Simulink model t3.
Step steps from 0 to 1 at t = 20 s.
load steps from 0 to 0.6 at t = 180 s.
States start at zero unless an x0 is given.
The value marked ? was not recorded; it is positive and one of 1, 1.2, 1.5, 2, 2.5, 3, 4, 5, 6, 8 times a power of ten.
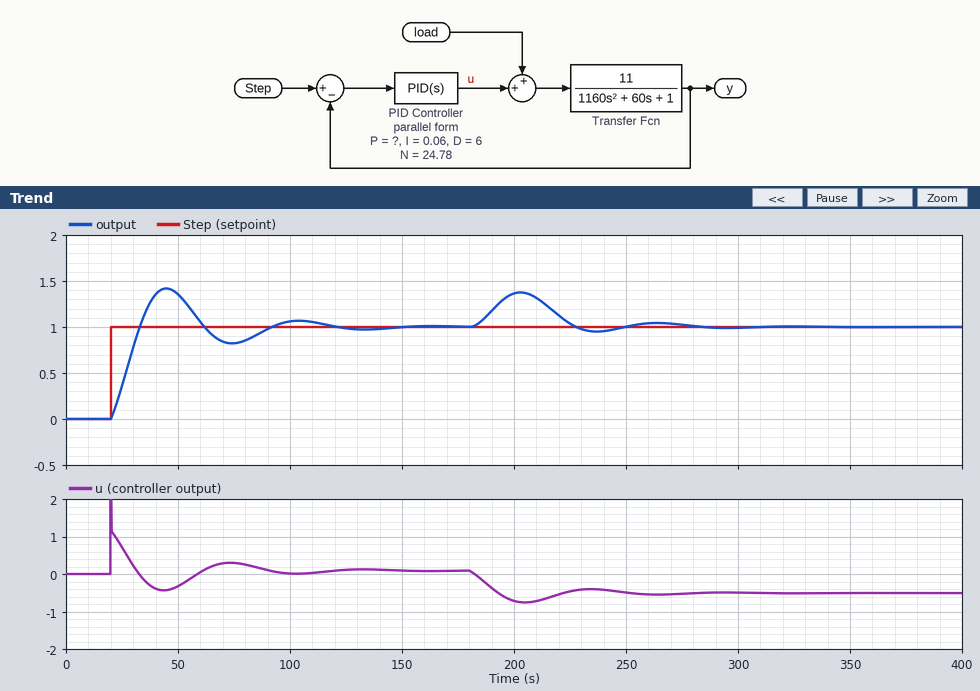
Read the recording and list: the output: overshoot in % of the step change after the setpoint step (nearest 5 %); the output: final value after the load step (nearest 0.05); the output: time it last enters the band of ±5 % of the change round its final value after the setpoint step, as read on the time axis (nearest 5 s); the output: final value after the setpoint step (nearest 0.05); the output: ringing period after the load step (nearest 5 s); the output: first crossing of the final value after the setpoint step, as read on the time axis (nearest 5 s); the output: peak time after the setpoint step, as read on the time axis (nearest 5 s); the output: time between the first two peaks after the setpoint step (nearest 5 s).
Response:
40 %
1.00
110 s
1.00
60 s
35 s
45 s
60 s
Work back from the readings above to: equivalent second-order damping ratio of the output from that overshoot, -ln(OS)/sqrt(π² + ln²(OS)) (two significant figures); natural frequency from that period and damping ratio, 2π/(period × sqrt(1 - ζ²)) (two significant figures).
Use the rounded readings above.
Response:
0.28
0.11 rad/s
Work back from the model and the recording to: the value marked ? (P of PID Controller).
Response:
1.5
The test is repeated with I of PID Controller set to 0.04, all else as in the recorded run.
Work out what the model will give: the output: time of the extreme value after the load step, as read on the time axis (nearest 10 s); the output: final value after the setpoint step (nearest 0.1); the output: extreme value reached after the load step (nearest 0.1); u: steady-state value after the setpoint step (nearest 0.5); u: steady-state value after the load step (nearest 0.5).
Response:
200 s
1.0
1.4
0.0
-0.5
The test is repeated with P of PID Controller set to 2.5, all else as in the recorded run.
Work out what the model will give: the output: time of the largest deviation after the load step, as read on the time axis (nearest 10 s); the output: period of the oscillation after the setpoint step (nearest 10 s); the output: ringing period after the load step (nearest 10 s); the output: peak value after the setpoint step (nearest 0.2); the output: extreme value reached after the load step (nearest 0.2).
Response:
200 s
40 s
40 s
1.4
1.2
